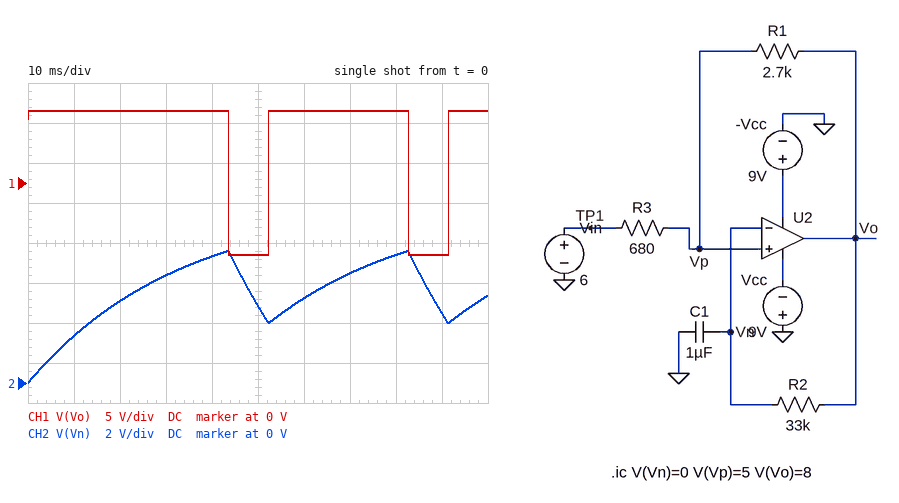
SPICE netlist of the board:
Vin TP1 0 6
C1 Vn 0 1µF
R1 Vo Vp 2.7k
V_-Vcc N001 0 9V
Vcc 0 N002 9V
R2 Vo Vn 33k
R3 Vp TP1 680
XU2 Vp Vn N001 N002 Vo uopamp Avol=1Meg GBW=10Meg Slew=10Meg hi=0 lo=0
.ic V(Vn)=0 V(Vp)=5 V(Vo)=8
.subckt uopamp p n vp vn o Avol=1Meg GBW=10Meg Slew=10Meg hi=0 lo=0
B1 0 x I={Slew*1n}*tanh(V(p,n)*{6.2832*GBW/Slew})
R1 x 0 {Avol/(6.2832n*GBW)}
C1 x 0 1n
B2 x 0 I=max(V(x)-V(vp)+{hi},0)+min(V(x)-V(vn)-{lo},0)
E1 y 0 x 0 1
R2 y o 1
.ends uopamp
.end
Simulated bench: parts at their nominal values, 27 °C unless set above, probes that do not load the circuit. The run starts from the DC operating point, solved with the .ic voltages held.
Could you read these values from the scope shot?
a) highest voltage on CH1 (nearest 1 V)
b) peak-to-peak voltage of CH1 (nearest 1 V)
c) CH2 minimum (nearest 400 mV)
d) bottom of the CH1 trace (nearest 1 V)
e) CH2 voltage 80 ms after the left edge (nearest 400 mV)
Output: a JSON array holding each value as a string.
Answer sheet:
["9 V", "18 V", "0 V", "-9 V", "6.4 V"]
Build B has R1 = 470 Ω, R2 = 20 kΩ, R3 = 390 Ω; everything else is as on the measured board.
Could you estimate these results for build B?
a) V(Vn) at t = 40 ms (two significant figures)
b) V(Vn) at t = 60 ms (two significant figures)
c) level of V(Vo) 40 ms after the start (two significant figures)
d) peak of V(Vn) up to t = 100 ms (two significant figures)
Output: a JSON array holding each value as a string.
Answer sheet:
["3.1 V", "3.7 V", "-9.0 V", "7.4 V"]
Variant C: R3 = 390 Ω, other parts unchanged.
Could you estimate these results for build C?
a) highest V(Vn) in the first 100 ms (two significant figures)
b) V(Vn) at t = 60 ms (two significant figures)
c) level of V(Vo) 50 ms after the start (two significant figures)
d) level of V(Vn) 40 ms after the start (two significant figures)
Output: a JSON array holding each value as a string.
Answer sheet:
["6.4 V", "5.8 V", "9.0 V", "6.3 V"]
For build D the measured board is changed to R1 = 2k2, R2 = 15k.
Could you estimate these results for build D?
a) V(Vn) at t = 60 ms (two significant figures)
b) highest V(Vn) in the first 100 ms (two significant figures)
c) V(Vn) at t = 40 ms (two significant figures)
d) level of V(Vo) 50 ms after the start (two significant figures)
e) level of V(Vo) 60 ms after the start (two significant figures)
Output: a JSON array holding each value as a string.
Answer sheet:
["6.5 V", "6.7 V", "6.6 V", "9.0 V", "9.0 V"]
